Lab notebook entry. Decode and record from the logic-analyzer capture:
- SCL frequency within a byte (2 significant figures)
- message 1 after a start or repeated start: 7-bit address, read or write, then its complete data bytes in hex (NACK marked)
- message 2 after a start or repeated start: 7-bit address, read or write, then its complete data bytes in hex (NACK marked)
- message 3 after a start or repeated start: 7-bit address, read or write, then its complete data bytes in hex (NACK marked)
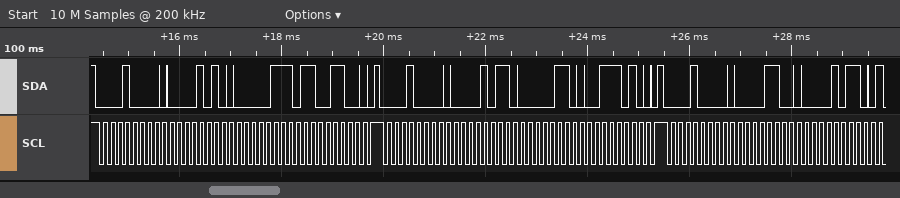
6.9 kHz
0x08 write: 0A 07 CC
0x08 write: 0B 06 3A
0x08 write: 0C 0B
